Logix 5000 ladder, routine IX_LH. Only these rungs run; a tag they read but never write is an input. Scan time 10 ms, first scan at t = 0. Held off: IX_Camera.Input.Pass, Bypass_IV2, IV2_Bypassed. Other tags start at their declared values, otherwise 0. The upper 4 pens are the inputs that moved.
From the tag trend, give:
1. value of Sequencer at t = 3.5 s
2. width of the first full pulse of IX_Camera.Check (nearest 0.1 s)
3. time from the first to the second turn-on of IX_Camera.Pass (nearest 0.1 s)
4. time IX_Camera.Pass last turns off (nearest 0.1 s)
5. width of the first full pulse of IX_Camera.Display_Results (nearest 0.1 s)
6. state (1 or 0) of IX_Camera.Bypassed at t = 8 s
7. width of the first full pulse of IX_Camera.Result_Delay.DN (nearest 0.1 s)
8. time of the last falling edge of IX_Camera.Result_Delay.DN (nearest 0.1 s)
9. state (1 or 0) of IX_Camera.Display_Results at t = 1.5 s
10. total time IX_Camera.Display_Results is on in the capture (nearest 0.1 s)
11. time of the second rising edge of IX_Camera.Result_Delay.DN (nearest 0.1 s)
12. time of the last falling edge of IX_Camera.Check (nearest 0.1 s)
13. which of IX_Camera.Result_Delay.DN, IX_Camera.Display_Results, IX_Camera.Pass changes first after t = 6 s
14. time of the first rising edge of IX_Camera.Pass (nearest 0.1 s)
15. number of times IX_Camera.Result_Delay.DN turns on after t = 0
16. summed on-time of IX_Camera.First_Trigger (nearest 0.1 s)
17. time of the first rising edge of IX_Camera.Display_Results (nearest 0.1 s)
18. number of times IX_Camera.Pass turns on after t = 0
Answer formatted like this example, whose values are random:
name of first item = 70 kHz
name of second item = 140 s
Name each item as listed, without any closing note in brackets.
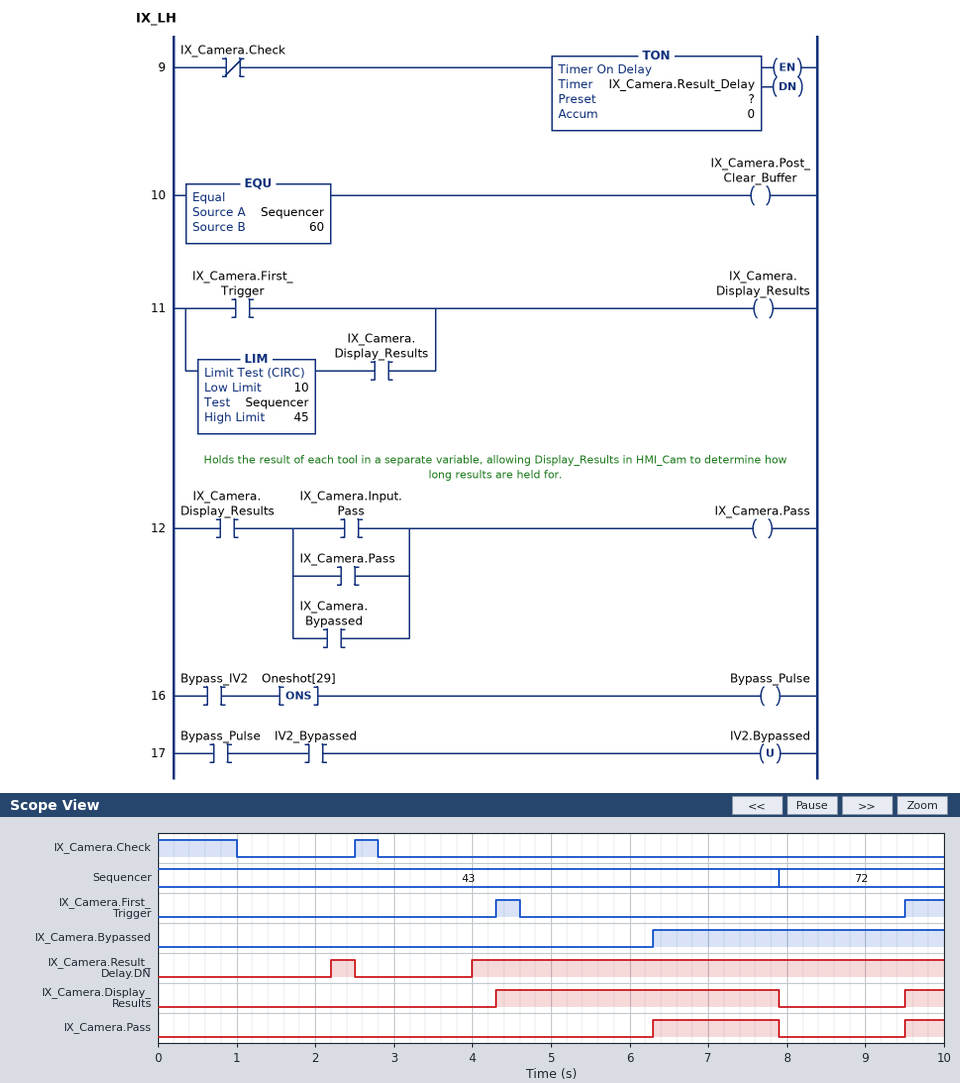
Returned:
value of Sequencer at t = 3.5 s = 43
width of the first full pulse of IX_Camera.Check = 0.3 s
time from the first to the second turn-on of IX_Camera.Pass = 3.2 s
time IX_Camera.Pass last turns off = 7.9 s
width of the first full pulse of IX_Camera.Display_Results = 3.6 s
state (1 or 0) of IX_Camera.Bypassed at t = 8 s = 1
width of the first full pulse of IX_Camera.Result_Delay.DN = 0.3 s
time of the last falling edge of IX_Camera.Result_Delay.DN = 2.5 s
state (1 or 0) of IX_Camera.Display_Results at t = 1.5 s = 0
total time IX_Camera.Display_Results is on in the capture = 4.1 s
time of the second rising edge of IX_Camera.Result_Delay.DN = 4.0 s
time of the last falling edge of IX_Camera.Check = 2.8 s
which of IX_Camera.Result_Delay.DN, IX_Camera.Display_Results, IX_Camera.Pass changes first after t = 6 s = IX_Camera.Pass
time of the first rising edge of IX_Camera.Pass = 6.3 s
number of times IX_Camera.Result_Delay.DN turns on after t = 0 = 2
summed on-time of IX_Camera.First_Trigger = 0.8 s
time of the first rising edge of IX_Camera.Display_Results = 4.3 s
number of times IX_Camera.Pass turns on after t = 0 = 2
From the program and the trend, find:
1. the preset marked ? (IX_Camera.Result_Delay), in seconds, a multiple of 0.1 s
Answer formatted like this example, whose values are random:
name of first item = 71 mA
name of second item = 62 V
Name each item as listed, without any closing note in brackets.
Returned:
the preset marked ? (IX_Camera.Result_Delay), in seconds, a multiple of 0.1 s = 1.2 s
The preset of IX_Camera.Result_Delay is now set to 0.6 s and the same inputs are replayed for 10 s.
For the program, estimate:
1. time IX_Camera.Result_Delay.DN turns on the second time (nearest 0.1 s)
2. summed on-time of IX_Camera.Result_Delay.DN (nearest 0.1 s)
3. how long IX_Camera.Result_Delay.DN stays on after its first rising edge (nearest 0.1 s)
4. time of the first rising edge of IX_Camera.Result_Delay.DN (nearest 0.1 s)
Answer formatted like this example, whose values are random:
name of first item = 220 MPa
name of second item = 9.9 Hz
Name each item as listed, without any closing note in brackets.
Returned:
time IX_Camera.Result_Delay.DN turns on the second time = 3.4 s
summed on-time of IX_Camera.Result_Delay.DN = 7.5 s
how long IX_Camera.Result_Delay.DN stays on after its first rising edge = 0.9 s
time of the first rising edge of IX_Camera.Result_Delay.DN = 1.6 s
